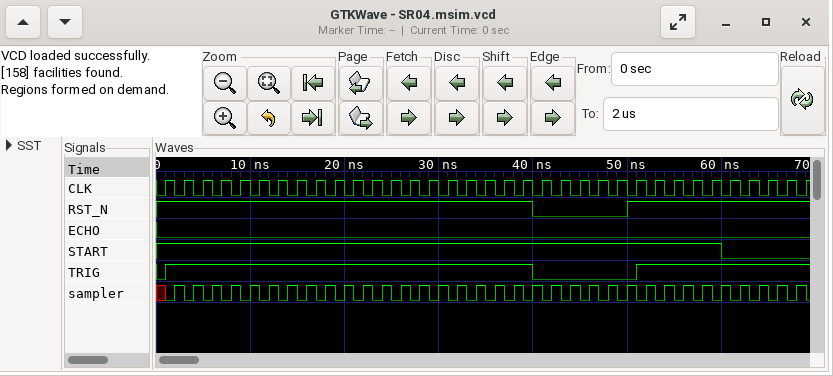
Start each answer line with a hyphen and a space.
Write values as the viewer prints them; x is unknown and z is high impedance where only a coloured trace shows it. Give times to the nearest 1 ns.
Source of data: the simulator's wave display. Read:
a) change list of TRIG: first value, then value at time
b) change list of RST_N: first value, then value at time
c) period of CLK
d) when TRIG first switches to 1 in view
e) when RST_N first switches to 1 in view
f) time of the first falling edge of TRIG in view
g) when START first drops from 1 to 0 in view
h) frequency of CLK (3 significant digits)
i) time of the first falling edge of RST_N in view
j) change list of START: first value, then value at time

- 0, 1 at 1 ns, 0 at 40 ns, 1 at 51 ns
- 1, 0 at 40 ns, 1 at 50 ns
- 2 ns
- 1 ns
- 50 ns
- 40 ns
- 60 ns
- 500 MHz
- 40 ns
- 1, 0 at 60 ns
